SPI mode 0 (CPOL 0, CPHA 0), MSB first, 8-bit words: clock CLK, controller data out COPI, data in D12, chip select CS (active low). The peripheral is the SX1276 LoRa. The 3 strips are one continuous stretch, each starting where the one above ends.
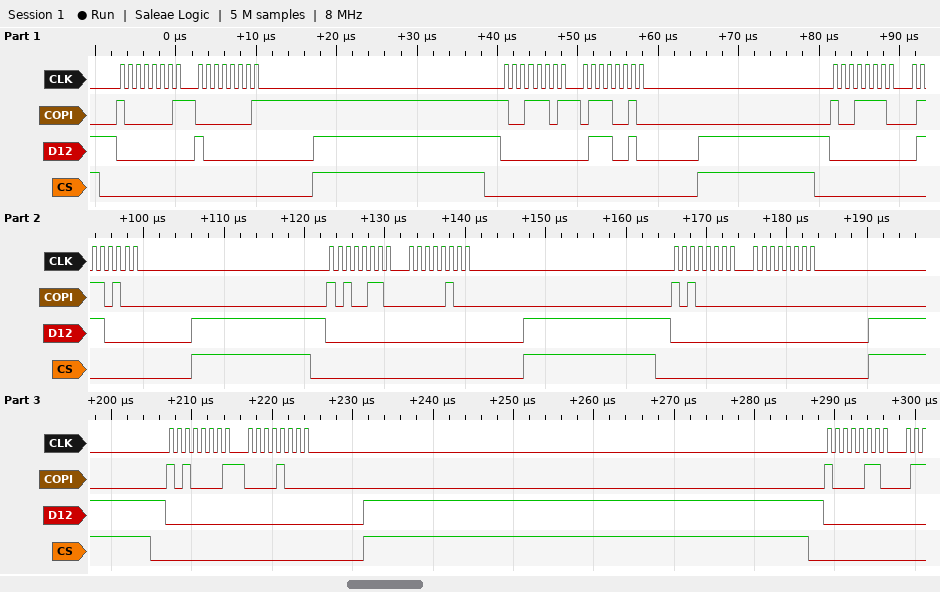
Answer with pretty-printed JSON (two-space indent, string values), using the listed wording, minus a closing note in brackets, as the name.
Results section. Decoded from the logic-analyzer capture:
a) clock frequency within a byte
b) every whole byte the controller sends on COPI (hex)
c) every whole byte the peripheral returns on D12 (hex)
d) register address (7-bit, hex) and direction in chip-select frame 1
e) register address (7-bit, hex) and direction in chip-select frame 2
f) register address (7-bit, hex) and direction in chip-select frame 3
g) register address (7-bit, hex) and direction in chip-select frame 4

{
  "clock frequency within a byte": "1 MHz",
  "every whole byte the controller sends on COPI": "0x81 0x01 0x9D 0x72 0x9E 0x74 0xA6 0x04 0xA0 0x00 0xA1 0x08 0x86",
  "every whole byte the peripheral returns on D12": "0x00 0x80 0x00 0x72 0x00 0x70 0x00 0x00 0x00 0x00 0x00 0x00 0x00",
  "register address (7-bit, hex) and direction in chip-select frame 1": "0x01 write",
  "register address (7-bit, hex) and direction in chip-select frame 2": "0x1D write",
  "register address (7-bit, hex) and direction in chip-select frame 3": "0x1E write",
  "register address (7-bit, hex) and direction in chip-select frame 4": "0x26 write"
}
